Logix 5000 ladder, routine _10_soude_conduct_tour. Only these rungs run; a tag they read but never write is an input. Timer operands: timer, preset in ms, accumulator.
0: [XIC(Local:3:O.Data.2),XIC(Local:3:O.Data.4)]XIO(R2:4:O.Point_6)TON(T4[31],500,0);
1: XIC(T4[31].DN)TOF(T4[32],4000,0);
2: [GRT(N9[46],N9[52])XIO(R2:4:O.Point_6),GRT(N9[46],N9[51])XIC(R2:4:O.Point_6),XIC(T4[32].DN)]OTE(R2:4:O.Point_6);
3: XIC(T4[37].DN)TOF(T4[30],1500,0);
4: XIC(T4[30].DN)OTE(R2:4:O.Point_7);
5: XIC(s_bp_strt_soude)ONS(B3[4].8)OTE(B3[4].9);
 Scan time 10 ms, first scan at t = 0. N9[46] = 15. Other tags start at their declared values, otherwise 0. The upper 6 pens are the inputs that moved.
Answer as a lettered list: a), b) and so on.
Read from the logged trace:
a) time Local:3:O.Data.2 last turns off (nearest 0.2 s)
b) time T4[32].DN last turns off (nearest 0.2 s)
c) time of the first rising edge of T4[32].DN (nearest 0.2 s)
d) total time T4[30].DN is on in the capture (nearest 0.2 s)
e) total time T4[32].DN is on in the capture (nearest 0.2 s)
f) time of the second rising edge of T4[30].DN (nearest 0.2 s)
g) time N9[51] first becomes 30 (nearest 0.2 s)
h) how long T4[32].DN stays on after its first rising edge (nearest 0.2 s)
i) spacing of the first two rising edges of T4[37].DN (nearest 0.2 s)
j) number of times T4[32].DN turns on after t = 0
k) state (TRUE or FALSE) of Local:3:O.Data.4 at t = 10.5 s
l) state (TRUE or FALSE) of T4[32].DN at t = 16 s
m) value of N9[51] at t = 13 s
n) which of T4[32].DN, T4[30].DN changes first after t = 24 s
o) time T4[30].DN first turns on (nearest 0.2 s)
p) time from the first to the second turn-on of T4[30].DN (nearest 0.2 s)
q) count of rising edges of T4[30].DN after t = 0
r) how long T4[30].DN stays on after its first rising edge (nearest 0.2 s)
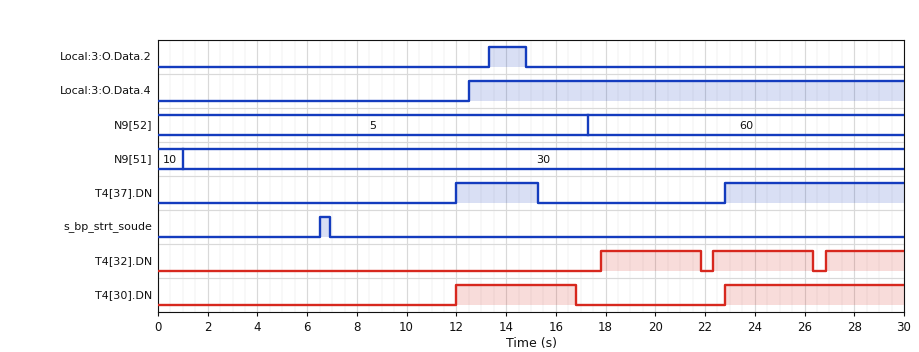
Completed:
a) 14.8 s
b) 26.4 s
c) 17.8 s
d) 12.0 s
e) 11.2 s
f) 22.8 s
g) 1.0 s
h) 4.0 s
i) 10.8 s
j) 3
k) FALSE
l) FALSE
m) 30
n) T4[32].DN
o) 12.0 s
p) 10.8 s
q) 2
r) 4.8 s
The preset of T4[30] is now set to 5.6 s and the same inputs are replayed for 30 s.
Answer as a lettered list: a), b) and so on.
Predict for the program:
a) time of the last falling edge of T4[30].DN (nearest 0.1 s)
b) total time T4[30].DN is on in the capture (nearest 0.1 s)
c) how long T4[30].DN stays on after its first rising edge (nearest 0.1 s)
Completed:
a) 20.9 s
b) 16.1 s
c) 8.9 s
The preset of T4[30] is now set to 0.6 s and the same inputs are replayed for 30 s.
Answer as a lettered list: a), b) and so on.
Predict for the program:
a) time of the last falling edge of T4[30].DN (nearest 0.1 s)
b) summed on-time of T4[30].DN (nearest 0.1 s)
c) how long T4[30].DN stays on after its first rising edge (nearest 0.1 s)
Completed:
a) 15.9 s
b) 11.1 s
c) 3.9 s
